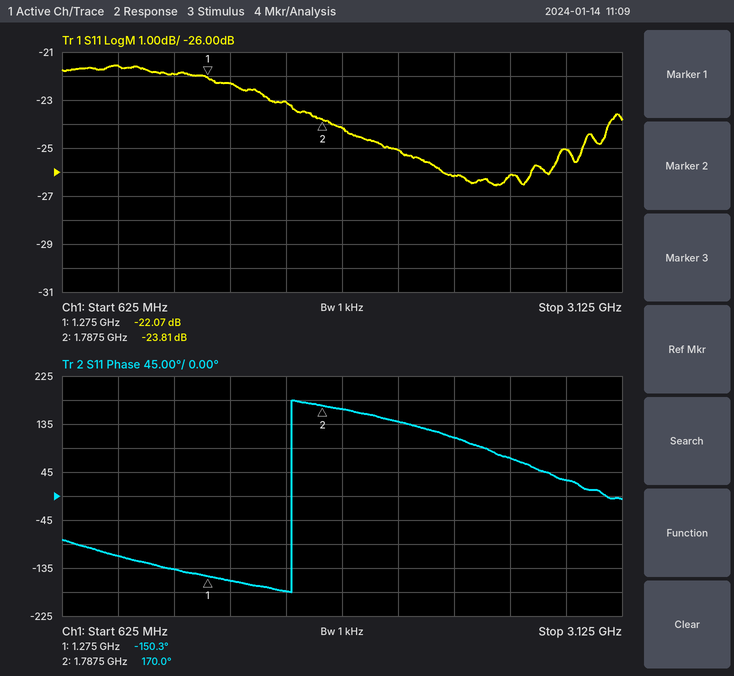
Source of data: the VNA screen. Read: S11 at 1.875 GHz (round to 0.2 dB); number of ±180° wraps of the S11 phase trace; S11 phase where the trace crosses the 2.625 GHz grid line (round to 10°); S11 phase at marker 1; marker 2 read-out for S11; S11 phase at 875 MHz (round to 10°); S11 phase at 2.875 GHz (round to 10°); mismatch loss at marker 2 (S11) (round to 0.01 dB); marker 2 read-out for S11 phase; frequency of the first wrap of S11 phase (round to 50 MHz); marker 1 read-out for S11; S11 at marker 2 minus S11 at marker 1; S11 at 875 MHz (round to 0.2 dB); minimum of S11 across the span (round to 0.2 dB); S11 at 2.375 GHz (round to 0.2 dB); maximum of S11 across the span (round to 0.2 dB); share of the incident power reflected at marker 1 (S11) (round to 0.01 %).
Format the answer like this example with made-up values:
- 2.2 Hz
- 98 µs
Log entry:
- -24.2 dB
- 1
- 70°
- -150.3°
- -23.81 dB
- -110°
- 30°
- 0.02 dB
- 170.0°
- 1.65 GHz
- -22.07 dB
- -1.74 dB
- -21.6 dB
- -26.6 dB
- -26.2 dB
- -21.6 dB
- 0.62 %
